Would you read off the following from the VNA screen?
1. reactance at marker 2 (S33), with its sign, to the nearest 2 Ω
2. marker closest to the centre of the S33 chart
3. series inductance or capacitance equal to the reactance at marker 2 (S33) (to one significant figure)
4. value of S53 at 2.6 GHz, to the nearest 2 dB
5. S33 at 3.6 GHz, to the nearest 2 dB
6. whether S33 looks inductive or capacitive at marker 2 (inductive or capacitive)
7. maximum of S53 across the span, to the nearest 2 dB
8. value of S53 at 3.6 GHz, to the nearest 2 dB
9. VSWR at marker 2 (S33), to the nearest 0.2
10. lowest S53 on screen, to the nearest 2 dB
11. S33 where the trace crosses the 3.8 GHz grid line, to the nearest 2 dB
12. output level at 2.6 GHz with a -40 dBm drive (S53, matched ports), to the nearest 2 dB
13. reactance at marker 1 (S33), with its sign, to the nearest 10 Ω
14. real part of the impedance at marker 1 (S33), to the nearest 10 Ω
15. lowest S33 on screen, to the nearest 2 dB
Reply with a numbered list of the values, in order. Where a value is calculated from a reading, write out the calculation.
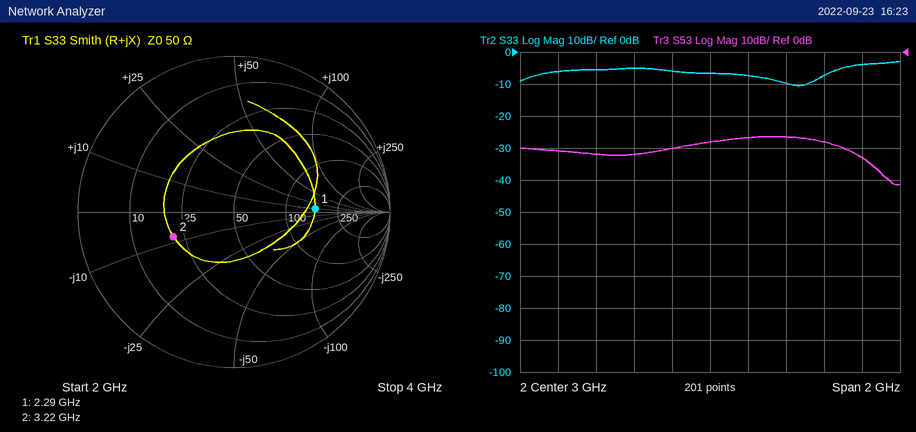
1. -8 Ω
2. marker 2
3. C = 1/(2π × 3.22 GHz × 8 Ω) ≈ 6 pF
4. -32 dB
5. -8 dB
6. capacitive
7. -26 dB
8. -28 dB
9. 2.4
10. -42 dB
11. -4 dB
12. -40 dBm + (-32 dB) = -72 dBm
13. +10 Ω
14. 160 Ω
15. -10 dB
